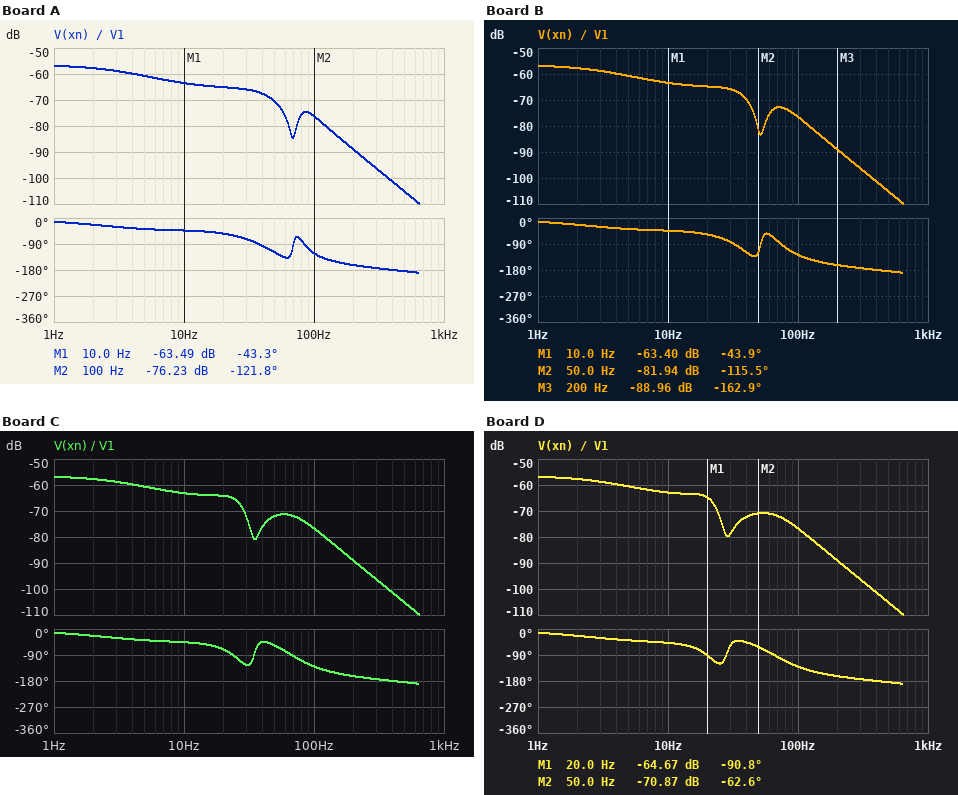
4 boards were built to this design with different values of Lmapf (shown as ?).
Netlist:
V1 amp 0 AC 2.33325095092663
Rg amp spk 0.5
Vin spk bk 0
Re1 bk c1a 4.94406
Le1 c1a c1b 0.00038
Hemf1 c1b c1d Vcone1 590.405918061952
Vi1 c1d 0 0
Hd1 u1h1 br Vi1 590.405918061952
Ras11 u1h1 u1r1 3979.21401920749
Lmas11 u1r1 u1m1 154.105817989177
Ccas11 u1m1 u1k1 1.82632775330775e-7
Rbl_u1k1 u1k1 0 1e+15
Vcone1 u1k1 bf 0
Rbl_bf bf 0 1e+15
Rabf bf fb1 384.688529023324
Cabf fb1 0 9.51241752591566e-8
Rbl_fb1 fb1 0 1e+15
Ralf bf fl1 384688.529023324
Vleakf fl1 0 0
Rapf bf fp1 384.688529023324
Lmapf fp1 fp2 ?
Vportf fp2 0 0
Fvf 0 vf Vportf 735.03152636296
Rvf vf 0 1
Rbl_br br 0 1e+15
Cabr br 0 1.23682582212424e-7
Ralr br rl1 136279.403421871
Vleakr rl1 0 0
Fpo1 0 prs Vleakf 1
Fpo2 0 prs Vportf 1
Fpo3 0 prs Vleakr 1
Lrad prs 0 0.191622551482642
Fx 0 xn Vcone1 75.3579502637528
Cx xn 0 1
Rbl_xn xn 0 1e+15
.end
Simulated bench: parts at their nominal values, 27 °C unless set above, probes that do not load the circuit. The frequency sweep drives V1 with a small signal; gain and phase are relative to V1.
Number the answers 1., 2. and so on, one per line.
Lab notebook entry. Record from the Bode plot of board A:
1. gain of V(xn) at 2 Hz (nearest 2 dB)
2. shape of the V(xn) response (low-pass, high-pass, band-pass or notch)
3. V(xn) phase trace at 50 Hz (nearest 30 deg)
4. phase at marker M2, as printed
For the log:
1. -58 dB
2. low-pass
3. -120 deg
4. -121.8 deg
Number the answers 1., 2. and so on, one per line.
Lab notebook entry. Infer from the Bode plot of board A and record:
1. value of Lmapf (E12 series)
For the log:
1. 56 H
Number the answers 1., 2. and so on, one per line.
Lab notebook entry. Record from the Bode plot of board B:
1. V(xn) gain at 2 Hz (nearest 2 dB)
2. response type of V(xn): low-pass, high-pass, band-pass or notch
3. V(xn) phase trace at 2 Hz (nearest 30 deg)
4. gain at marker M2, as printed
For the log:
1. -58 dB
2. low-pass
3. -30 deg
4. -81.94 dB
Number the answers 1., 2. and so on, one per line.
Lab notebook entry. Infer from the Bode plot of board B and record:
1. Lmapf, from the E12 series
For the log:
1. 100 H
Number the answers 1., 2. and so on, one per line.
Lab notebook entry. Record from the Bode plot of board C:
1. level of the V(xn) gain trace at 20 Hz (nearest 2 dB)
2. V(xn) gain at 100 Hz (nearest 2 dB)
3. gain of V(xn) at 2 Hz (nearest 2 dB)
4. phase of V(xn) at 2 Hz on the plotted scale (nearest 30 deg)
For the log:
1. -64 dB
2. -76 dB
3. -58 dB
4. -30 deg
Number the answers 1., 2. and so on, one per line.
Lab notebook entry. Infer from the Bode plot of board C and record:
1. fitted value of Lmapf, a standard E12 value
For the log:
1. 220 H
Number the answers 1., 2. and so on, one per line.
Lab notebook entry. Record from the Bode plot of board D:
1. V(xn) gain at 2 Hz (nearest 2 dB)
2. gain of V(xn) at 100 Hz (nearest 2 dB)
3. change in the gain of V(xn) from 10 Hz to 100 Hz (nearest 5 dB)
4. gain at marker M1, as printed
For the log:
1. -58 dB
2. -76 dB
3. -15 dB
4. -64.67 dB
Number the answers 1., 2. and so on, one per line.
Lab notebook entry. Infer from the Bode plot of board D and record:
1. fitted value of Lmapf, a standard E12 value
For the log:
1. 330 H
